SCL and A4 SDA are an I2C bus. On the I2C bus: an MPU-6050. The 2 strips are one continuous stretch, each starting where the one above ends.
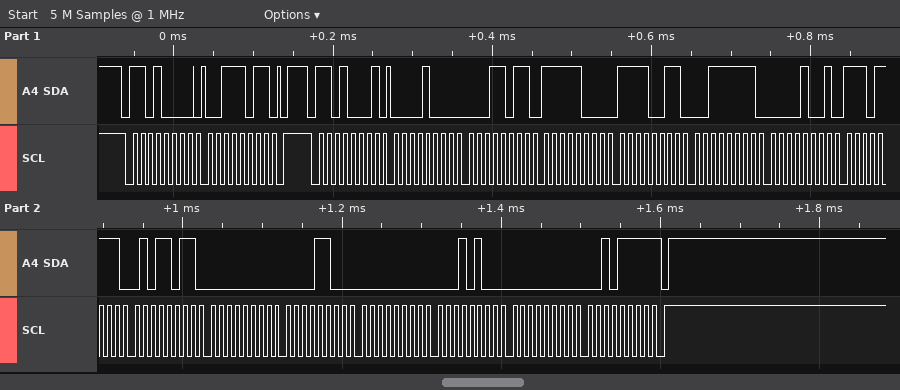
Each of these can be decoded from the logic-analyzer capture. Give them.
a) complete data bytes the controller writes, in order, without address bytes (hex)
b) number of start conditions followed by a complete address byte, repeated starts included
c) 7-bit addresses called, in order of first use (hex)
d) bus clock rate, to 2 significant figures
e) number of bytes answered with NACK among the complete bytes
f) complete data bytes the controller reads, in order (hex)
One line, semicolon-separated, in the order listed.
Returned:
3B; 2; 0x68; 100 kHz; 1; 08 1B F8 F3 3F 09 EF 5B 00 0C 00 14 00 2F
